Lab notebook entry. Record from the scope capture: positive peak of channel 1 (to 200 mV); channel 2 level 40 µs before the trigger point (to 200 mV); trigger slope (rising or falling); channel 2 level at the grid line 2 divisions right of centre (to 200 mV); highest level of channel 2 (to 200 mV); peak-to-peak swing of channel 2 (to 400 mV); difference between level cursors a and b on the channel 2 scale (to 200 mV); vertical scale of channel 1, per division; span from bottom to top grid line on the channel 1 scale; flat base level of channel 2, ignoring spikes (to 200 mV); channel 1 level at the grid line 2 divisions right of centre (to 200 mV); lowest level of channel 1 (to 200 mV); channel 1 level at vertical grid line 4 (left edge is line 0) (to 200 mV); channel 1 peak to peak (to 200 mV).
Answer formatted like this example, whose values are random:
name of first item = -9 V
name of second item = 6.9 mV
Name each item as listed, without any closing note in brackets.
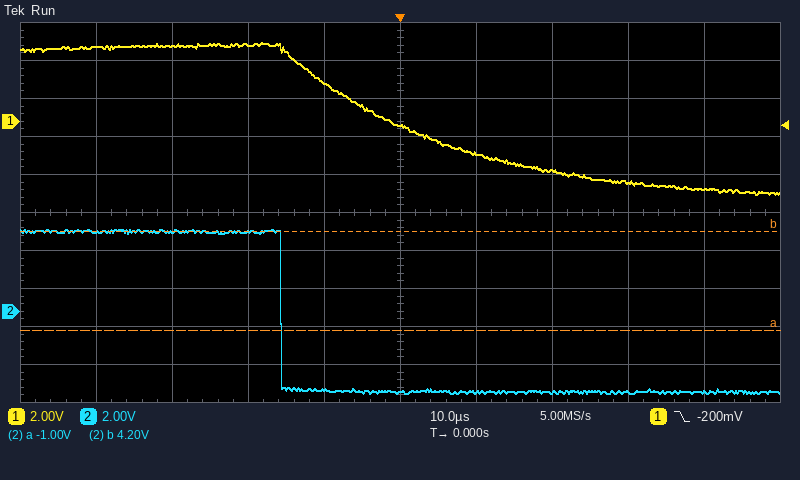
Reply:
positive peak of channel 1 = 4.2 V
channel 2 level 40 µs before the trigger point = 4.2 V
trigger slope = falling
channel 2 level at the grid line 2 divisions right of centre = -4.2 V
highest level of channel 2 = 4.4 V
peak-to-peak swing of channel 2 = 8.8 V
difference between level cursors a and b on the channel 2 scale = 5.2 V
vertical scale of channel 1, per division = 2 V
span from bottom to top grid line on the channel 1 scale = 20 V
flat base level of channel 2, ignoring spikes = -4.2 V
channel 1 level at the grid line 2 divisions right of centre = -2.6 V
lowest level of channel 1 = -3.8 V
channel 1 level at vertical grid line 4 (left edge is line 0) = 2.0 V
channel 1 peak to peak = 8.0 V
